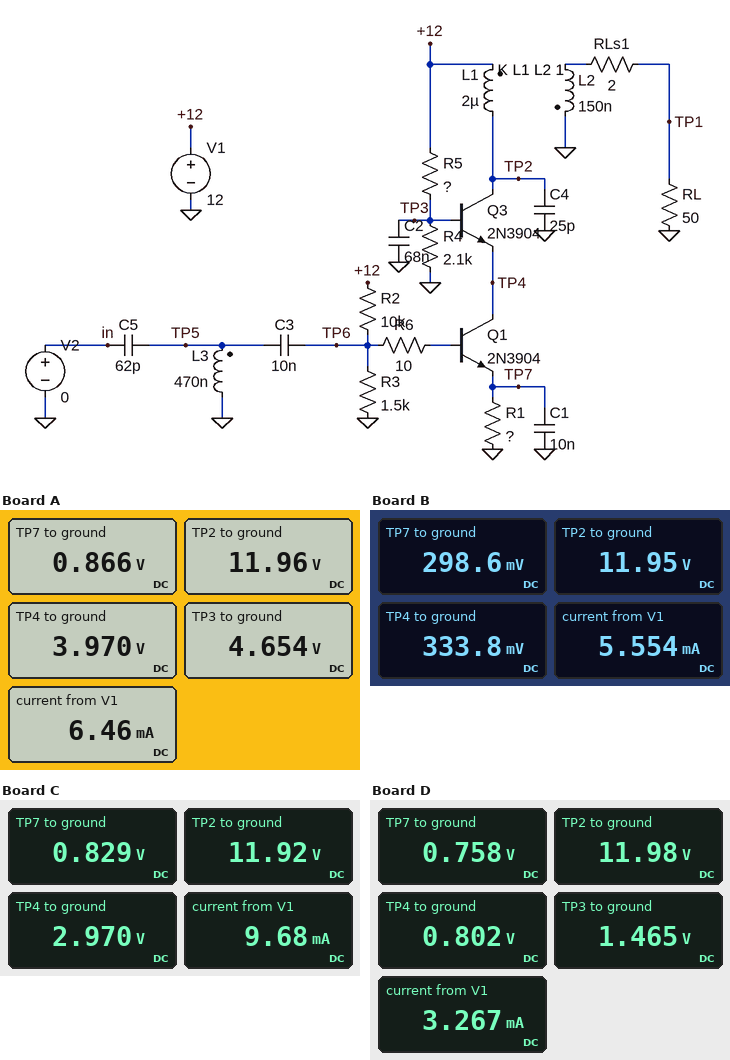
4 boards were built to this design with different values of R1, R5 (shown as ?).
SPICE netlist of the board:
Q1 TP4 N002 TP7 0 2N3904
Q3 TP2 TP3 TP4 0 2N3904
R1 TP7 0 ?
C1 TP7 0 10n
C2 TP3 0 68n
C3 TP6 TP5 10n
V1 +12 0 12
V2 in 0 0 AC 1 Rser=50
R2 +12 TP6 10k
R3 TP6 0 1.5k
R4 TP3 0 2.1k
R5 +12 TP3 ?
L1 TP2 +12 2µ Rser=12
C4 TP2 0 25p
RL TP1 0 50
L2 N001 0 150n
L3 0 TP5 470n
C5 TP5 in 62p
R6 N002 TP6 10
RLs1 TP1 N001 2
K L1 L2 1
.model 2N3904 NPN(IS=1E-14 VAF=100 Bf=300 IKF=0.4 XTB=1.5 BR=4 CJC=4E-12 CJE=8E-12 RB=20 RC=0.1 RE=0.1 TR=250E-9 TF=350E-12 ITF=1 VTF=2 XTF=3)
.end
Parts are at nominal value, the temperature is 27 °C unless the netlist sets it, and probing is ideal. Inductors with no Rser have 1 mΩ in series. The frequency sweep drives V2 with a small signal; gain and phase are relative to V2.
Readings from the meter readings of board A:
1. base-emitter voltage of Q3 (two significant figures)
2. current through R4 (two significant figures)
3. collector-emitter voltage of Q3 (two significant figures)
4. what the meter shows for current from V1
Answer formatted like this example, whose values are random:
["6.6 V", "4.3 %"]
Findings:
["680 mV", "2.2 mA", "8.0 V", "6.46 mA"]
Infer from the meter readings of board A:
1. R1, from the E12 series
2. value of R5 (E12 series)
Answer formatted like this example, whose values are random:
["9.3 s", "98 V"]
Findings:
["270 Ω", "3.3 kΩ"]
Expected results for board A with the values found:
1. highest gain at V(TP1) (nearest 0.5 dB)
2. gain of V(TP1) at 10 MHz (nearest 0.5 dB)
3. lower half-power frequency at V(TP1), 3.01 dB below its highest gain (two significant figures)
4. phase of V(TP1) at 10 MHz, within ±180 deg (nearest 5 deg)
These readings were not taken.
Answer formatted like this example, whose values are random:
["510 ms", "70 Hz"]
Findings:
["29.0 dB", "-3.0 dB", "19 MHz", "65 deg"]
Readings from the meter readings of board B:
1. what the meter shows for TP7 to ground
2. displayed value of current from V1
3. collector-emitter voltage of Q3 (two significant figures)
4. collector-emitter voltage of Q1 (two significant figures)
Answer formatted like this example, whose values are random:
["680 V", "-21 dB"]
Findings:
["298.6 mV", "5.554 mA", "12 V", "35 mV"]
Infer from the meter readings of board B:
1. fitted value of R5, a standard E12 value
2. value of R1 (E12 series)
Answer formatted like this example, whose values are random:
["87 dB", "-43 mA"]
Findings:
["22 kΩ", "68 Ω"]
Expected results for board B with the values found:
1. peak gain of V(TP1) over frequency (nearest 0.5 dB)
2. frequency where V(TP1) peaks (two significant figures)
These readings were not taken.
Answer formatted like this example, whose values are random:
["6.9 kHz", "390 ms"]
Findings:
["-7.5 dB", "21 MHz"]
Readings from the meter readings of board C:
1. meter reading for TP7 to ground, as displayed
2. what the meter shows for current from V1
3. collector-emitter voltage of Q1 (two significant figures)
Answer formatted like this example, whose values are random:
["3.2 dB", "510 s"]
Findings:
["0.829 V", "9.68 mA", "2.1 V"]
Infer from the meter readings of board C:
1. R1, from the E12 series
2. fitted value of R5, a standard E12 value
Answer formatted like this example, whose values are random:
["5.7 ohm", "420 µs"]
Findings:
["120 Ω", "4.7 kΩ"]
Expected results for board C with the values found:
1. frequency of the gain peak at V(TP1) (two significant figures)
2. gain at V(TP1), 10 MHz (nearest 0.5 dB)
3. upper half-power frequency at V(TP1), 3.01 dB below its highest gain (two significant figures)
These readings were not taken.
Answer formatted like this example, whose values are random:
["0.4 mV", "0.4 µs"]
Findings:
["19 MHz", "4.0 dB", "23 MHz"]
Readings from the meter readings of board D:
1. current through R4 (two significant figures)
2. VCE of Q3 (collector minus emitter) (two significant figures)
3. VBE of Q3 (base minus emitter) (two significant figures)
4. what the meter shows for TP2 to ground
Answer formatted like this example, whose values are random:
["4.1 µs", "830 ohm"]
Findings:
["700 µA", "11 V", "660 mV", "11.98 V"]
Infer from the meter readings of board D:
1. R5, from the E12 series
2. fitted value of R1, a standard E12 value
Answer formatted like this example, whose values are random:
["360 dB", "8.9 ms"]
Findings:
["15 kΩ", "470 Ω"]
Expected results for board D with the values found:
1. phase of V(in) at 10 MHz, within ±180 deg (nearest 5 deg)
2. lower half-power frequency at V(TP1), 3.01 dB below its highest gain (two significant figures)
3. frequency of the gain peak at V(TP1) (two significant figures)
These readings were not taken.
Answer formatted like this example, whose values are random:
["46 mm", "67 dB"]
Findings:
["-10 deg", "18 MHz", "22 MHz"]
